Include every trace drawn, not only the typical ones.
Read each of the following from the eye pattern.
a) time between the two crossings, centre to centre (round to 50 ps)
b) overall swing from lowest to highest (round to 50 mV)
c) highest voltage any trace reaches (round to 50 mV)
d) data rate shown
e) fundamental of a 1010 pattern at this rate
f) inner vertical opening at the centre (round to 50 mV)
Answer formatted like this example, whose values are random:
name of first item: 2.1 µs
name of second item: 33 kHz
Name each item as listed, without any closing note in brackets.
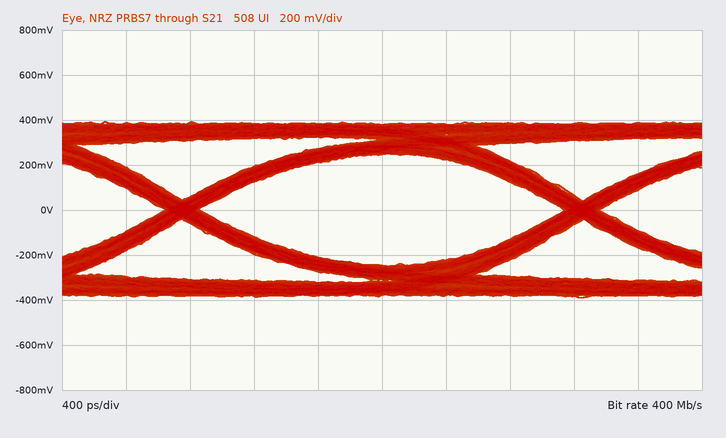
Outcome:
time between the two crossings, centre to centre: 2.50 ns
overall swing from lowest to highest: 800 mV
highest voltage any trace reaches: 400 mV
data rate shown: 400 Mb/s
fundamental of a 1010 pattern at this rate: 200 MHz
inner vertical opening at the centre: 500 mV
